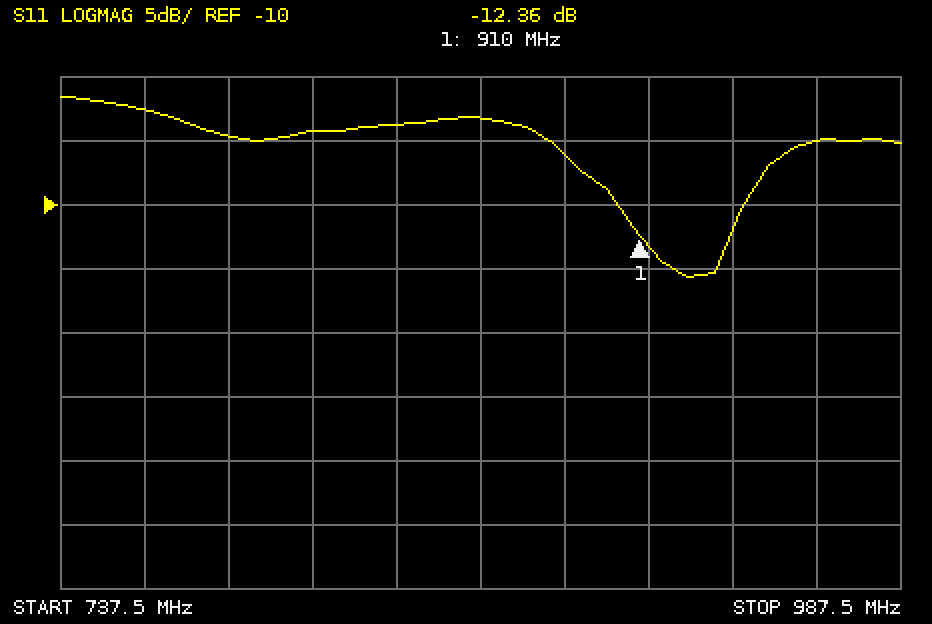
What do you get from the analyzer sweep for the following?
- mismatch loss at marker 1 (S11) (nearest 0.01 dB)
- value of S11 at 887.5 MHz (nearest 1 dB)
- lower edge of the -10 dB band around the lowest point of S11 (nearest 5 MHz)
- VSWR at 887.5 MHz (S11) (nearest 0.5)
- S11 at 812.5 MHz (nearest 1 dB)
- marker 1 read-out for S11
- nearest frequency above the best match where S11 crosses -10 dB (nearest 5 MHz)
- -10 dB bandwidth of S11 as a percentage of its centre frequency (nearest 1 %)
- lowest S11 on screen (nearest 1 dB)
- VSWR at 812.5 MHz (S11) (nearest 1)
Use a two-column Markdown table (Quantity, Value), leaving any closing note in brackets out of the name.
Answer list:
| Quantity | Value |
|---|---|
| mismatch loss at marker 1 (S11) | 0.26 dB |
| value of S11 at 887.5 MHz | -6 dB |
| lower edge of the -10 dB band around the lowest point of S11 | 905 MHz |
| VSWR at 887.5 MHz (S11) | 3.0 |
| S11 at 812.5 MHz | -4 dB |
| marker 1 read-out for S11 | -12.36 dB |
| nearest frequency above the best match where S11 crosses -10 dB | 940 MHz |
| -10 dB bandwidth of S11 as a percentage of its centre frequency | 4 % |
| lowest S11 on screen | -16 dB |
| VSWR at 812.5 MHz (S11) | 4 |
